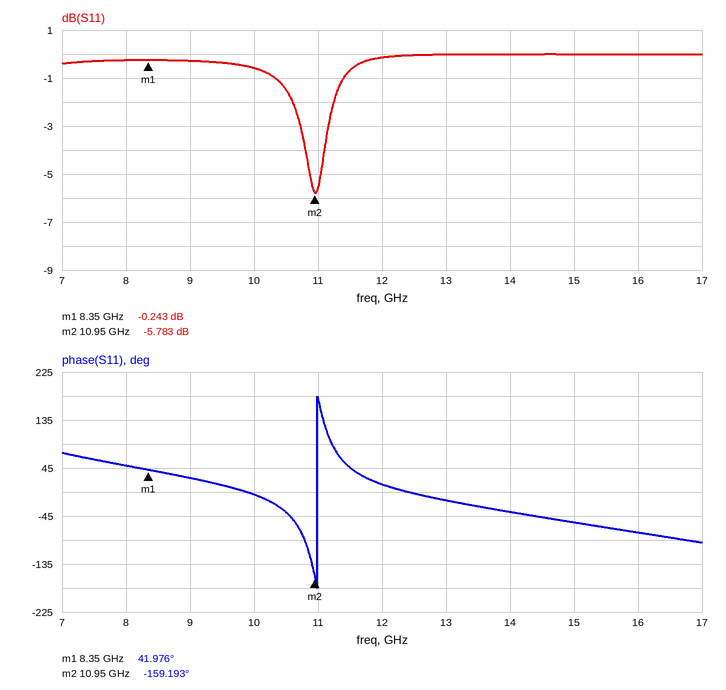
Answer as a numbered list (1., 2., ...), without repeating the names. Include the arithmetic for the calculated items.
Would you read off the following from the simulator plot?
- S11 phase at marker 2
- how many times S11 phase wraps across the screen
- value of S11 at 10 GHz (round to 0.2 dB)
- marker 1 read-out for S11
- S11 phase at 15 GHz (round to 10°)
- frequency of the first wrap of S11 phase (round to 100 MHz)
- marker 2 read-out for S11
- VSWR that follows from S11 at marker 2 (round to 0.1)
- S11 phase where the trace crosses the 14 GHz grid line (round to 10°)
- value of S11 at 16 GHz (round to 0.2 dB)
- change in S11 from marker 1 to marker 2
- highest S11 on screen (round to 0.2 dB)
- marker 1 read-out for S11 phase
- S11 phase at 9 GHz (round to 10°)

1. -159.193°
2. 1
3. -0.6 dB
4. -0.243 dB
5. -60°
6. 11.0 GHz
7. -5.783 dB
8. (1 + 0.5139)/(1 − 0.5139) ≈ 3.1
9. -40°
10. 0.0 dB
11. -5.783 − (-0.243) = -5.540 dB
12. 0.0 dB
13. 41.976°
14. 30°
